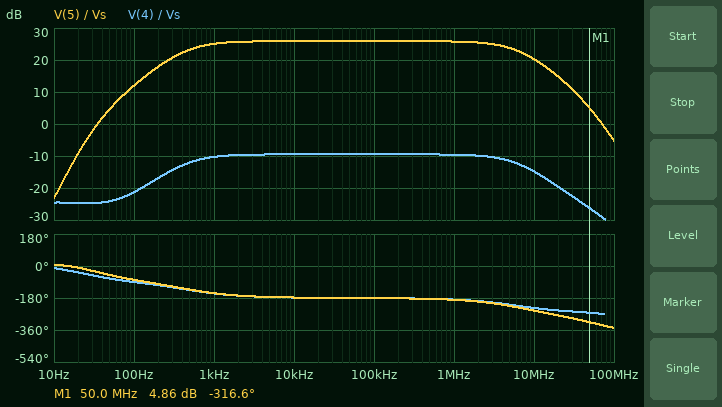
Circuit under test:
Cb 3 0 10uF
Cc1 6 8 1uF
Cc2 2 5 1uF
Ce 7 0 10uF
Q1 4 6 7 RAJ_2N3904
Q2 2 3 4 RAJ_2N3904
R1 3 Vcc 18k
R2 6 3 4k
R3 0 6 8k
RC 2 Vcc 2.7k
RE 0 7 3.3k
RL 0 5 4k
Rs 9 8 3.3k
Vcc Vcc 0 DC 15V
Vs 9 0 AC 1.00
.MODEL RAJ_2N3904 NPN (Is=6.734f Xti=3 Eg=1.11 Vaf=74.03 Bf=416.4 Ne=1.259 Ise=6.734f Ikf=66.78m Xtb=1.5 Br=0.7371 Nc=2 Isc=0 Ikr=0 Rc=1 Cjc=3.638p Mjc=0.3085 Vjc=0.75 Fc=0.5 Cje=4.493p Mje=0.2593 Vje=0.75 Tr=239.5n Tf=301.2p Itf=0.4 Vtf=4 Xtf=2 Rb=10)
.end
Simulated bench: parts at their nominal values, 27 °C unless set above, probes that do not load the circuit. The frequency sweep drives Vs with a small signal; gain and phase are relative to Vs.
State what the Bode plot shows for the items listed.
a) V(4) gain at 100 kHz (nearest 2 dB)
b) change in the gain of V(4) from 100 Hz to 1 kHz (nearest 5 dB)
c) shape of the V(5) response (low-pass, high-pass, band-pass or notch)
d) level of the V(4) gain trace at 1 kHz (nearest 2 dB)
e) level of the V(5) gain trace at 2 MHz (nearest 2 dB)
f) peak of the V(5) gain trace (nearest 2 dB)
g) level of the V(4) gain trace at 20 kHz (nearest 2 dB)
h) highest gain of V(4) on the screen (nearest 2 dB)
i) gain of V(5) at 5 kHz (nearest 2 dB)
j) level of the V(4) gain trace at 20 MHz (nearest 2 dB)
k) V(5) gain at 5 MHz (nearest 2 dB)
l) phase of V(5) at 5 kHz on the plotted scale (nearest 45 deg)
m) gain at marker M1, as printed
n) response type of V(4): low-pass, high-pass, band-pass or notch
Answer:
-10 dB
10 dB
band-pass
-10 dB
26 dB
26 dB
-10 dB
-10 dB
26 dB
-20 dB
24 dB
-180 deg
4.86 dB
band-pass
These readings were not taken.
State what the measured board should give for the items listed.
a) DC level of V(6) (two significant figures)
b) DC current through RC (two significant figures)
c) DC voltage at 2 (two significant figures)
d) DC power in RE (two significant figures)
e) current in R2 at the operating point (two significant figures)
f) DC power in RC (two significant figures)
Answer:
3.9 V
970 µA
12 V
3.2 mW
500 µA
2.6 mW
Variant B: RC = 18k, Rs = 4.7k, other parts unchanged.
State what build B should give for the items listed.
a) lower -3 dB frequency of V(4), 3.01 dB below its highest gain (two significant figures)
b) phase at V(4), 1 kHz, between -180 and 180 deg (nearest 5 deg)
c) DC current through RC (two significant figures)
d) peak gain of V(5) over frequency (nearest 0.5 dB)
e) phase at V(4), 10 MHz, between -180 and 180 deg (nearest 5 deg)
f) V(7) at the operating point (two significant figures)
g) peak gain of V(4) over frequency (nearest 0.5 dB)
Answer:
330 Hz
-165 deg
600 µA
2.5 dB
115 deg
2.5 V
-6.5 dB
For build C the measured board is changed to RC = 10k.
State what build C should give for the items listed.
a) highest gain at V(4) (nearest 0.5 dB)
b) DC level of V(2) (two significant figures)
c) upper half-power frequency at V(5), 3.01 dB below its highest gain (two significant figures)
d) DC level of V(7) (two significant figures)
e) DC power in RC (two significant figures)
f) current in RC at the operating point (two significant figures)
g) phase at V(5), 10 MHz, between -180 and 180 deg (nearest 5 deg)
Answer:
-7.0 dB
5.4 V
2.2 MHz
3.2 V
9.3 mW
960 µA
45 deg
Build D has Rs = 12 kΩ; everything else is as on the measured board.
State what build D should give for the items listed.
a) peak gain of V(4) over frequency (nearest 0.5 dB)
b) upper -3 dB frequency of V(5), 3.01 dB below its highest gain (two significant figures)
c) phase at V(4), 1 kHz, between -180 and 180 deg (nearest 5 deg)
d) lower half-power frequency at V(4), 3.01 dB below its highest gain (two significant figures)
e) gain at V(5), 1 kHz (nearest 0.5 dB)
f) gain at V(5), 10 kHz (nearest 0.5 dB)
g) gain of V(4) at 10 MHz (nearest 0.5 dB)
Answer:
-18.5 dB
4.8 MHz
-160 deg
390 Hz
16.5 dB
17.0 dB
-25.5 dB
